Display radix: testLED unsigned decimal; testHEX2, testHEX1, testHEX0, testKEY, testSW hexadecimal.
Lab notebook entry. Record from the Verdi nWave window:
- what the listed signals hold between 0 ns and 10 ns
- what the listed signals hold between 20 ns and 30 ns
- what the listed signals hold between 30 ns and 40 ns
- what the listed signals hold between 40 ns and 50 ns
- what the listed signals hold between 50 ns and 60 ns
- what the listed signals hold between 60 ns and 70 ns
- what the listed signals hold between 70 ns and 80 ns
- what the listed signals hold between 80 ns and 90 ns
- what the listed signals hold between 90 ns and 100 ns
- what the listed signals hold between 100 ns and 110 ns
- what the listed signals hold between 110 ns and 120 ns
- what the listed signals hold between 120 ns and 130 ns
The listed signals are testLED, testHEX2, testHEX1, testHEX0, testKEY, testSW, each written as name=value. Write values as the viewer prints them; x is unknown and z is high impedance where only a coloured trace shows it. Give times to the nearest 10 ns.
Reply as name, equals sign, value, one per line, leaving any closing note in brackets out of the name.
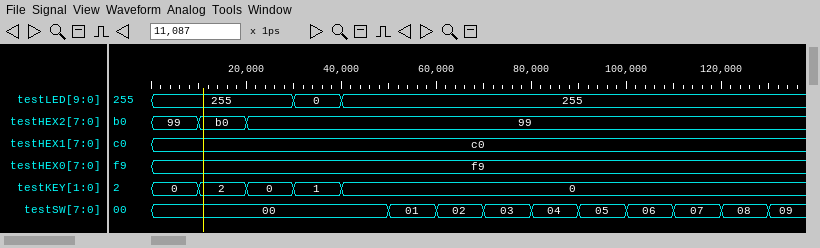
what the listed signals hold between 0 ns and 10 ns = testLED=255, testHEX2=99, testHEX1=c0, testHEX0=f9, testKEY=0, testSW=00
what the listed signals hold between 20 ns and 30 ns = testLED=255, testHEX2=99, testHEX1=c0, testHEX0=f9, testKEY=0, testSW=00
what the listed signals hold between 30 ns and 40 ns = testLED=0, testHEX2=99, testHEX1=c0, testHEX0=f9, testKEY=1, testSW=00
what the listed signals hold between 40 ns and 50 ns = testLED=255, testHEX2=99, testHEX1=c0, testHEX0=f9, testKEY=0, testSW=00
what the listed signals hold between 50 ns and 60 ns = testLED=255, testHEX2=99, testHEX1=c0, testHEX0=f9, testKEY=0, testSW=01
what the listed signals hold between 60 ns and 70 ns = testLED=255, testHEX2=99, testHEX1=c0, testHEX0=f9, testKEY=0, testSW=02
what the listed signals hold between 70 ns and 80 ns = testLED=255, testHEX2=99, testHEX1=c0, testHEX0=f9, testKEY=0, testSW=03
what the listed signals hold between 80 ns and 90 ns = testLED=255, testHEX2=99, testHEX1=c0, testHEX0=f9, testKEY=0, testSW=04
what the listed signals hold between 90 ns and 100 ns = testLED=255, testHEX2=99, testHEX1=c0, testHEX0=f9, testKEY=0, testSW=05
what the listed signals hold between 100 ns and 110 ns = testLED=255, testHEX2=99, testHEX1=c0, testHEX0=f9, testKEY=0, testSW=06
what the listed signals hold between 110 ns and 120 ns = testLED=255, testHEX2=99, testHEX1=c0, testHEX0=f9, testKEY=0, testSW=07
what the listed signals hold between 120 ns and 130 ns = testLED=255, testHEX2=99, testHEX1=c0, testHEX0=f9, testKEY=0, testSW=08
